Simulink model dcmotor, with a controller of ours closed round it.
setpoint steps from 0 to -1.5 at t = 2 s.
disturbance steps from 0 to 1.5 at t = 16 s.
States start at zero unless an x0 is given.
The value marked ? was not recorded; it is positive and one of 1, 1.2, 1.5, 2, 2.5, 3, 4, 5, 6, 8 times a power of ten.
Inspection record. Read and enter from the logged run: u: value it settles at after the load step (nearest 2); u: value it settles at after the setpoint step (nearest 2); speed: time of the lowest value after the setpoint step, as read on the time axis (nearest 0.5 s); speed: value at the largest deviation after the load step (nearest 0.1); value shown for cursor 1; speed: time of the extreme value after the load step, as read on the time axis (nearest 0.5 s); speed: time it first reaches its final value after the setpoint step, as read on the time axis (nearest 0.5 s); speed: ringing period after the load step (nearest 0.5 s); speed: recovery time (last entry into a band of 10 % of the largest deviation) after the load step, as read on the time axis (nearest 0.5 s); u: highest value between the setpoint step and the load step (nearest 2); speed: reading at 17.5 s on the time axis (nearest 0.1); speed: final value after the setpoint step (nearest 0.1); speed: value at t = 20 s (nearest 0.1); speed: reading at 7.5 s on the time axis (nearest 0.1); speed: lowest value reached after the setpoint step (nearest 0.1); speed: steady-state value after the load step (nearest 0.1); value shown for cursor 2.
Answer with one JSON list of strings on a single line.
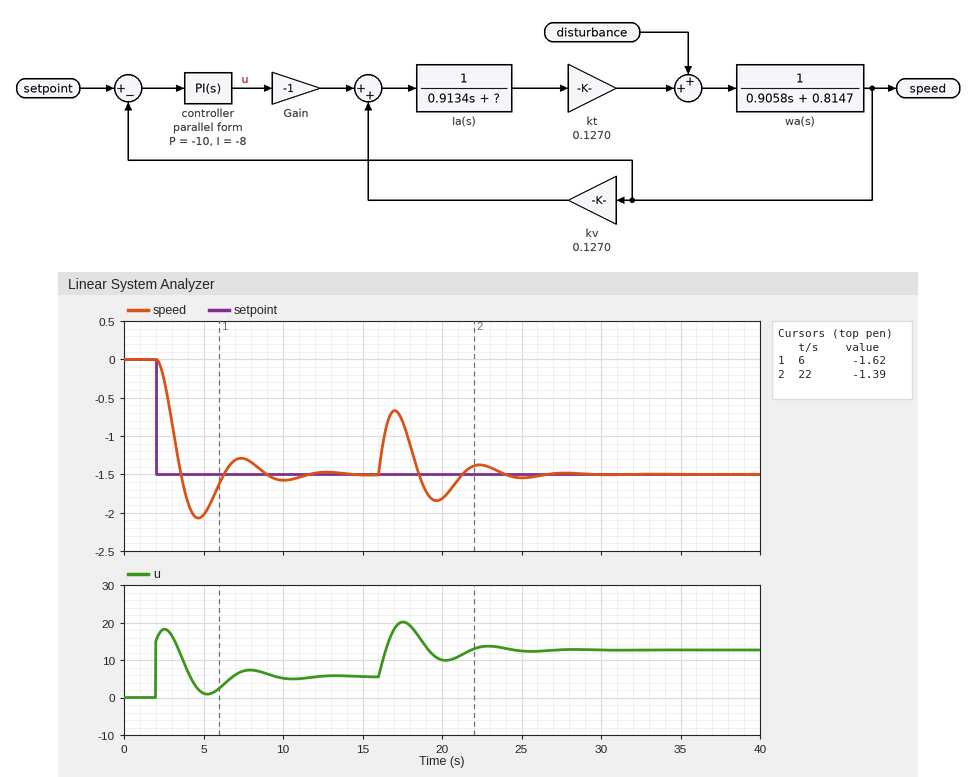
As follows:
["12", "6", "4.5 s", "-0.7", "-1.62", "17.0 s", "3.5 s", "5.5 s", "23.0 s", "18", "-0.8", "-1.5", "-1.8", "-1.3", "-2.1", "-1.5", "-1.39"]
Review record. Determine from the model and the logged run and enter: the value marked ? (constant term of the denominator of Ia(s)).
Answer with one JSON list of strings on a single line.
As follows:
["0.6"]
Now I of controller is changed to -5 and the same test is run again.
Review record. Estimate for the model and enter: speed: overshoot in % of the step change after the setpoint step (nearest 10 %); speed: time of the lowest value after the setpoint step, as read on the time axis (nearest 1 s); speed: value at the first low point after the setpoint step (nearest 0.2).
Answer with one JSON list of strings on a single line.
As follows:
["20 %", "5 s", "-1.8"]
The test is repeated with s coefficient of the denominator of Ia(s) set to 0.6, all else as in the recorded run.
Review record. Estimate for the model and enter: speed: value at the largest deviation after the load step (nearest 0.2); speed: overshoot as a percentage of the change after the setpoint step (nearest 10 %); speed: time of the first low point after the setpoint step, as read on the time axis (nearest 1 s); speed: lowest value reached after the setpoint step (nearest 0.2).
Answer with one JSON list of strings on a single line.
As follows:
["-0.8", "30 %", "4 s", "-2.0"]
